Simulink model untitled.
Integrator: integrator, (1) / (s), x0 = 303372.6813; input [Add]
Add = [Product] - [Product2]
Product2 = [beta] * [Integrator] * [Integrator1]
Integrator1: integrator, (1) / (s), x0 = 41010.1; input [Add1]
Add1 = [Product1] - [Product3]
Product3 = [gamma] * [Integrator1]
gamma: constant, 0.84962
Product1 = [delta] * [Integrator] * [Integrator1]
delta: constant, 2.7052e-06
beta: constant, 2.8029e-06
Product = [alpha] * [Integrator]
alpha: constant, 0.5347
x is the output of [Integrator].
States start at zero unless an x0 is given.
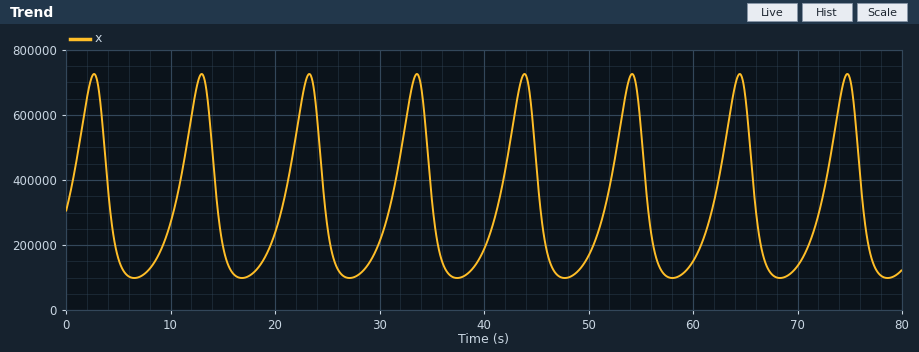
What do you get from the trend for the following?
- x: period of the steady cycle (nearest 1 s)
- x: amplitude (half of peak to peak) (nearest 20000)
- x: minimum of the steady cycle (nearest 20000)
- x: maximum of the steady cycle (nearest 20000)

10 s
320000
100000
720000
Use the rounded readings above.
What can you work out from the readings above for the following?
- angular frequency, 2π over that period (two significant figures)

0.63 rad/s
